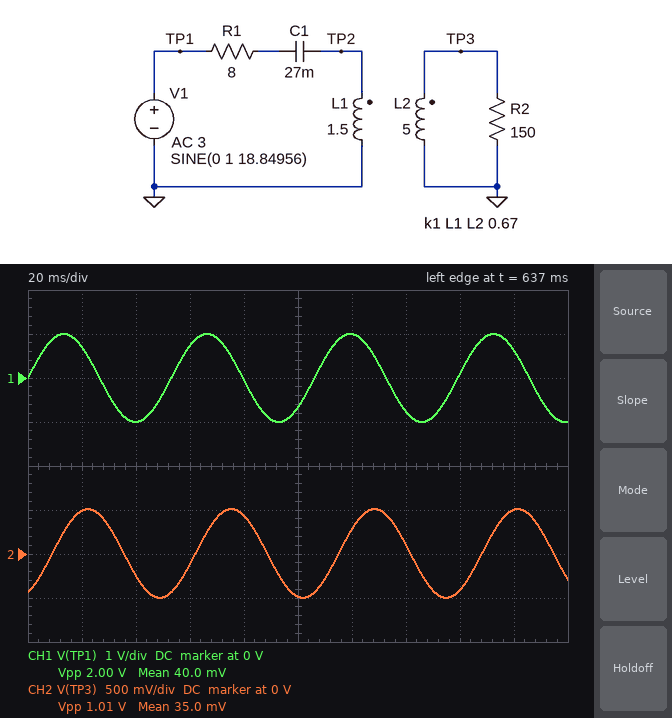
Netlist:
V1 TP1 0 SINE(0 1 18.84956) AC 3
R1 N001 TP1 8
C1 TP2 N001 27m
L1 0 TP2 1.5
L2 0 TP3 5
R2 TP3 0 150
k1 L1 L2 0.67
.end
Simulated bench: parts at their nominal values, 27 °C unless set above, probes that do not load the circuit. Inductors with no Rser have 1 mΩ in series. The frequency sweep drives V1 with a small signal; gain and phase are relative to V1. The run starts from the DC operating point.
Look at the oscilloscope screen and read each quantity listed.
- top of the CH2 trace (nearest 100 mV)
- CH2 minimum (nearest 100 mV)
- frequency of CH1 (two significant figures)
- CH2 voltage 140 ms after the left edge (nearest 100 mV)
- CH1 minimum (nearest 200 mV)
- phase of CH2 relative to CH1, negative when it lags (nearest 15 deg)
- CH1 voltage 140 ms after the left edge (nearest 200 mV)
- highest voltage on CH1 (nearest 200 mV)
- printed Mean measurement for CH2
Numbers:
500 mV
-500 mV
19 Hz
100 mV
-1.0 V
-60 deg
-800 mV
1.0 V
35.0 mV
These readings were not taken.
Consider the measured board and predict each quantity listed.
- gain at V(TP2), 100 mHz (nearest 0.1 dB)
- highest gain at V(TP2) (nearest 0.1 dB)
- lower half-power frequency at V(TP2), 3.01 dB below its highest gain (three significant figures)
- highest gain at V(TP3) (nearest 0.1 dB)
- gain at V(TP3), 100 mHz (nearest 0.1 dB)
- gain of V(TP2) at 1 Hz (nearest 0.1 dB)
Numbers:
-35.9 dB
0 dB
666 mHz
1.7 dB
-34.1 dB
-0.2 dB
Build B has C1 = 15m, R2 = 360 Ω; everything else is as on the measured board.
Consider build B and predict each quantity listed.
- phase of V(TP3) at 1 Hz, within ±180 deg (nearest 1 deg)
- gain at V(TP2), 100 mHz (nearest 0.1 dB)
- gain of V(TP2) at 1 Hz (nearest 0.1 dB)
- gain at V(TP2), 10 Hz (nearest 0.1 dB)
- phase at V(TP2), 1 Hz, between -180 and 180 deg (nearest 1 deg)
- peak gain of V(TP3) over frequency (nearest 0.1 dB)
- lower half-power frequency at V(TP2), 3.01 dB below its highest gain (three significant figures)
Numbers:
93 deg
-41.0 dB
0.9 dB
-0.2 dB
96 deg
3.9 dB
879 mHz
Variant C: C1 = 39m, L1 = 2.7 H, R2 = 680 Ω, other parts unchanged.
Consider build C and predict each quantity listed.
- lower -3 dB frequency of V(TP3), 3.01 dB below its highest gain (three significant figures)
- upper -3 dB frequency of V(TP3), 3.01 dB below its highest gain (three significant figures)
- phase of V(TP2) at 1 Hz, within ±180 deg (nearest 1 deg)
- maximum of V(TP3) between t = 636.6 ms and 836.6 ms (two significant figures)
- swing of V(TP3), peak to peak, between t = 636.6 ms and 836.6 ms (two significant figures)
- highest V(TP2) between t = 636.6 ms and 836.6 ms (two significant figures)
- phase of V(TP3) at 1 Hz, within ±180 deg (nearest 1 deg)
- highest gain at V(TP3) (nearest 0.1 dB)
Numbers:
416 mHz
26.1 Hz
32 deg
820 mV
1.6 V
990 mV
30 deg
0.6 dB
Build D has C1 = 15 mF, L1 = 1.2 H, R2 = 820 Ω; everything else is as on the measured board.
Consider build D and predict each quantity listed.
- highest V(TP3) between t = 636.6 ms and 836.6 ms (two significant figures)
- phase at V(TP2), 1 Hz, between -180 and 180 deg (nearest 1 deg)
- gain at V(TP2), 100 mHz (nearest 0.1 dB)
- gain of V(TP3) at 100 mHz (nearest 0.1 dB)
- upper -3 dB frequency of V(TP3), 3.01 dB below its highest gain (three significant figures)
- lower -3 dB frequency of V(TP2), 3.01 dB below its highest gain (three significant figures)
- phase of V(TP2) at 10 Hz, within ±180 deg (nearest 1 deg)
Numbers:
1.3 V
110 deg
-42.9 dB
-40.2 dB
26.9 Hz
995 mHz
6 deg
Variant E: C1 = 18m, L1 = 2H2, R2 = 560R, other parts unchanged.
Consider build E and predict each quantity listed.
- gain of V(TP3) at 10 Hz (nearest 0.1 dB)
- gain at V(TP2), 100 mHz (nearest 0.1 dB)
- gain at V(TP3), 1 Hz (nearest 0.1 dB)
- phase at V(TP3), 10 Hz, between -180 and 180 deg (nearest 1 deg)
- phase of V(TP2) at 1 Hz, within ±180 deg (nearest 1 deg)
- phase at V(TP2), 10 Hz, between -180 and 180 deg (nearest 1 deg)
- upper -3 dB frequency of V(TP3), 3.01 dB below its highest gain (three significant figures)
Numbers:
-0.4 dB
-36.0 dB
3.1 dB
-14 deg
58 deg
4 deg
3.62 Hz
